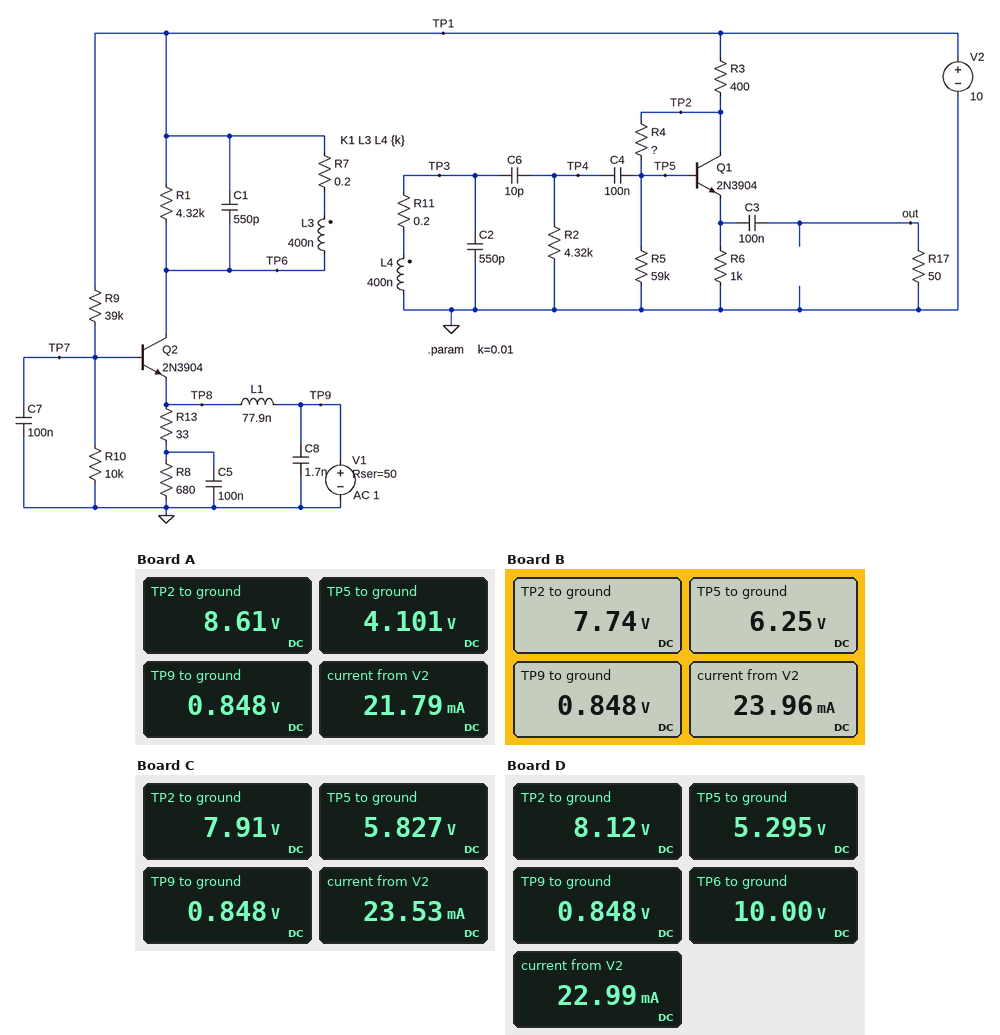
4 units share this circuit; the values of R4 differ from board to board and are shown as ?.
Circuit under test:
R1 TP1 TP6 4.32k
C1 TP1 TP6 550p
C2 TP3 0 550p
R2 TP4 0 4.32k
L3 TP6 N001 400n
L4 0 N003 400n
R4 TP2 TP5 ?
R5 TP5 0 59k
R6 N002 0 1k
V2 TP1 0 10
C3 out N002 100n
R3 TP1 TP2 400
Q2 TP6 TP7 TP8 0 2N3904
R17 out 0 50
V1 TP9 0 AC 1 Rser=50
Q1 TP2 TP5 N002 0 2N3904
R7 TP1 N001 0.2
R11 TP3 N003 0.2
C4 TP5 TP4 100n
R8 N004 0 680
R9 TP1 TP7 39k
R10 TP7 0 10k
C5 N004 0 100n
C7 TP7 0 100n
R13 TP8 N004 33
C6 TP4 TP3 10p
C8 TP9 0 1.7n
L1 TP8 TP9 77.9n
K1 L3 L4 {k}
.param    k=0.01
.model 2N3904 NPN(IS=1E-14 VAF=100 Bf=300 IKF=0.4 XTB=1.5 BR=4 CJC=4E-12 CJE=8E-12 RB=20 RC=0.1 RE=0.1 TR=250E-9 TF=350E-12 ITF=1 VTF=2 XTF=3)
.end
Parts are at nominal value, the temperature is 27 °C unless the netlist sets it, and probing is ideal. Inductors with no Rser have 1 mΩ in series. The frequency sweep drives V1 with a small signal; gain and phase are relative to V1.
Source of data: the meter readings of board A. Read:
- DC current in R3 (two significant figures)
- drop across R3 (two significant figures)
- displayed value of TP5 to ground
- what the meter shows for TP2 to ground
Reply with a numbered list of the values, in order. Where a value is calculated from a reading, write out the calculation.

1. (10 V - 8.61 V) / 400 Ω = 3.5 mA
2. 10 V - 8.61 V = 1.4 V
3. 4.101 V
4. 8.61 V
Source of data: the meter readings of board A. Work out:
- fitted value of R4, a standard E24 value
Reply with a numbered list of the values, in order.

1. 56 kΩ
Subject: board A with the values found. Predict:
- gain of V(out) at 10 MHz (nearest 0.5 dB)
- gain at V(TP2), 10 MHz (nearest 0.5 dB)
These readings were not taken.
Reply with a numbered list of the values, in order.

1. -16.5 dB
2. 1.5 dB
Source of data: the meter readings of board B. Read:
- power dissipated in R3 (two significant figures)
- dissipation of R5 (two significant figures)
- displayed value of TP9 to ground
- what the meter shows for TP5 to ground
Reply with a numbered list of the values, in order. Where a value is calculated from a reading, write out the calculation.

1. (10 V - 7.74 V)^2 / 400 Ω = 13 mW
2. (6.25 V)^2 / 59 kΩ = 660 µW
3. 0.848 V
4. 6.25 V
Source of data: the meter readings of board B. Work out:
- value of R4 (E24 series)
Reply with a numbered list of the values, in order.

1. 12 kΩ
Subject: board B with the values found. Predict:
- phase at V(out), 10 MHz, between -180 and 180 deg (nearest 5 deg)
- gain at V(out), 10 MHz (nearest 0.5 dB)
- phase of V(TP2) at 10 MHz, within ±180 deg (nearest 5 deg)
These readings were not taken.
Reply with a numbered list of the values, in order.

1. -105 deg
2. -18.0 dB
3. 70 deg
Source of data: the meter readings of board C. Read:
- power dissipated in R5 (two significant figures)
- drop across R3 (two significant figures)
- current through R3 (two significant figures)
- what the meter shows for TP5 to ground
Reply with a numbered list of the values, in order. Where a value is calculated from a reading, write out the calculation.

1. (5.827 V)^2 / 59 kΩ = 580 µW
2. 10 V - 7.91 V = 2.1 V
3. (10 V - 7.91 V) / 400 Ω = 5.2 mA
4. 5.827 V
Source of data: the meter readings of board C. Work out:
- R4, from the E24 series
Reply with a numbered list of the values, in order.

1. 18 kΩ
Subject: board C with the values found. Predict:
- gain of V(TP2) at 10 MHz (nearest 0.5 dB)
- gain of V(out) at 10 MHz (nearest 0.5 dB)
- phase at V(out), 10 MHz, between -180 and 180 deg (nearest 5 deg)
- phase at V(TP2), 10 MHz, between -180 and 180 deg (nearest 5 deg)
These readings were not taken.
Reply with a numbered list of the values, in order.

1. 1.0 dB
2. -17.5 dB
3. -110 deg
4. 65 deg
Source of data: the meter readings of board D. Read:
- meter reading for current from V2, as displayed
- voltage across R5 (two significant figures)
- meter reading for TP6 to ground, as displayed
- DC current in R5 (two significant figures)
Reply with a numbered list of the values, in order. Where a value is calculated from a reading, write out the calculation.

1. 22.99 mA
2. 5.295 V = 5.3 V
3. 10.00 V
4. (5.295 V) / 59 kΩ = 90 µA
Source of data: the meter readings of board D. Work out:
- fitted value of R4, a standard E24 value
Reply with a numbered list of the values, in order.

1. 27 kΩ
